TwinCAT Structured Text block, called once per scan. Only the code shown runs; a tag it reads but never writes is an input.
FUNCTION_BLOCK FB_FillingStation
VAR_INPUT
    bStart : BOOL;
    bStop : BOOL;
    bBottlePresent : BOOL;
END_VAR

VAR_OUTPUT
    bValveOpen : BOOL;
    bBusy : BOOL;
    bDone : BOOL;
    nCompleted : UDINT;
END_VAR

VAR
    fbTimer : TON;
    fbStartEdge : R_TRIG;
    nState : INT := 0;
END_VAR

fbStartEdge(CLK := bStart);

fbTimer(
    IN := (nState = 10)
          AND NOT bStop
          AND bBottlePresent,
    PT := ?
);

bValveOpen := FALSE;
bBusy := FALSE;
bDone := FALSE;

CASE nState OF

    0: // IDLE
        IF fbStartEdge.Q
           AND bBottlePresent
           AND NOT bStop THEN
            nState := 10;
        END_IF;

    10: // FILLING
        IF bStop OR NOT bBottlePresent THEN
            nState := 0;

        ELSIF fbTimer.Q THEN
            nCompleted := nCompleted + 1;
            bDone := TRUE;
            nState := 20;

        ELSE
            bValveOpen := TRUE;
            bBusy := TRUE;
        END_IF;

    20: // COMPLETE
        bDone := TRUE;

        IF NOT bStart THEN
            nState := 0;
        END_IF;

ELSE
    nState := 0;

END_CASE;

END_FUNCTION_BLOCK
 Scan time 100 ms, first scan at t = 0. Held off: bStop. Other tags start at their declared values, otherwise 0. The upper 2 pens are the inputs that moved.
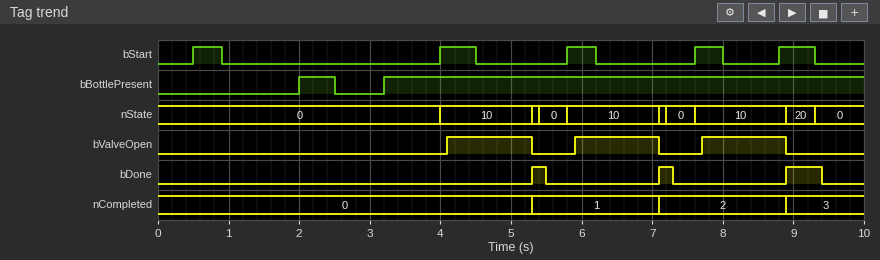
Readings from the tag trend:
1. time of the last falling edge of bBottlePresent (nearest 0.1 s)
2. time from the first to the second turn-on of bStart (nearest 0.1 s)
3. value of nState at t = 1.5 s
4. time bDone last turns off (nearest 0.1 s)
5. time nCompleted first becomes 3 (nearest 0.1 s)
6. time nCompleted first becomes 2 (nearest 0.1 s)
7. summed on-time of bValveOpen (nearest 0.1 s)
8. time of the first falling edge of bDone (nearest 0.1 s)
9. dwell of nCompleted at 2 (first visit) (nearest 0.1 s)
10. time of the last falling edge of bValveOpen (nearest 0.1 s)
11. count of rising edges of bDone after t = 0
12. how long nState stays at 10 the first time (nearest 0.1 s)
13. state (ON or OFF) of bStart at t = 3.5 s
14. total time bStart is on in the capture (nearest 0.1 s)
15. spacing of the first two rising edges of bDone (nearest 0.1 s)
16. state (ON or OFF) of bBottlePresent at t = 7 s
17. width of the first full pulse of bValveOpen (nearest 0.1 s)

2.5 s
3.5 s
0
9.4 s
8.9 s
7.1 s
3.6 s
5.5 s
1.8 s
8.9 s
3
1.3 s
OFF
2.2 s
1.8 s
ON
1.2 s
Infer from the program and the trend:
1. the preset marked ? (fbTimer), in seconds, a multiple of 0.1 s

1.2 s
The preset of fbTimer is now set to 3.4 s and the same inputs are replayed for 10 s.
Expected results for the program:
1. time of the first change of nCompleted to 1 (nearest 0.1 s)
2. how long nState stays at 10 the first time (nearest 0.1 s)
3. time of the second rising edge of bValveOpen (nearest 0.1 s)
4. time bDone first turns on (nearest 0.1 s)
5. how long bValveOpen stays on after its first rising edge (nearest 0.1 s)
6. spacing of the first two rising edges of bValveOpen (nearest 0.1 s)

7.5 s
3.5 s
8.9 s
7.5 s
3.4 s
4.8 s
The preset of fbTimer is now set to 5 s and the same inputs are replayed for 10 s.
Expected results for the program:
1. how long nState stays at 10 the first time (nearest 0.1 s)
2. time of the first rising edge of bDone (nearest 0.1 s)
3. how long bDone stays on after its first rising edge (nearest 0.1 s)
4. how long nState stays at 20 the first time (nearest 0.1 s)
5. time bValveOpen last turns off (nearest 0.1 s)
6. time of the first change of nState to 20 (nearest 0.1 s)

5.1 s
9.1 s
0.3 s
0.2 s
9.1 s
9.1 s
